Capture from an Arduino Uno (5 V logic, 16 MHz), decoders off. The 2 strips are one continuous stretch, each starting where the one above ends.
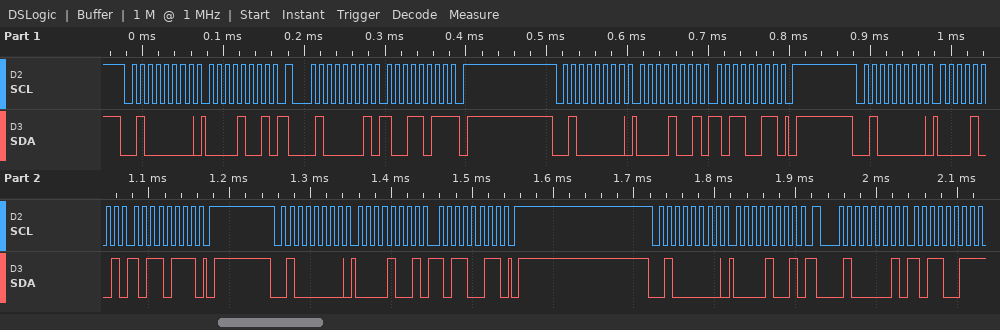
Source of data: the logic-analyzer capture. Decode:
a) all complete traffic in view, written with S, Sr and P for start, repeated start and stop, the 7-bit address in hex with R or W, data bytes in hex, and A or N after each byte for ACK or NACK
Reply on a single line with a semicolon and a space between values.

S 20W A 09 A Sr 20R A 9B N P S 20W A 09 A B3 A P S 20W A 09 A B7 A P S 20W A 09 A B3 A P S 20W A 09 A Sr 20R A B3 N
